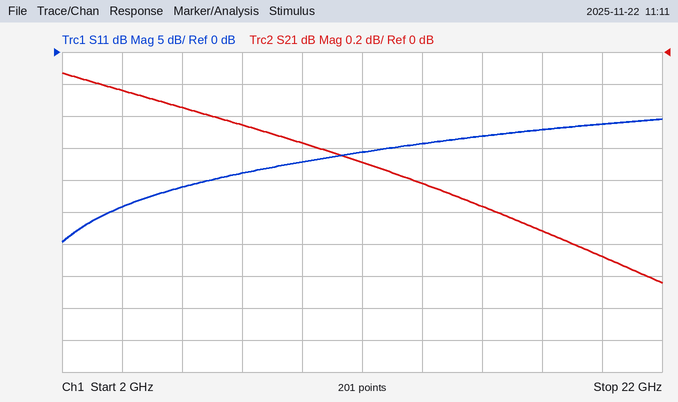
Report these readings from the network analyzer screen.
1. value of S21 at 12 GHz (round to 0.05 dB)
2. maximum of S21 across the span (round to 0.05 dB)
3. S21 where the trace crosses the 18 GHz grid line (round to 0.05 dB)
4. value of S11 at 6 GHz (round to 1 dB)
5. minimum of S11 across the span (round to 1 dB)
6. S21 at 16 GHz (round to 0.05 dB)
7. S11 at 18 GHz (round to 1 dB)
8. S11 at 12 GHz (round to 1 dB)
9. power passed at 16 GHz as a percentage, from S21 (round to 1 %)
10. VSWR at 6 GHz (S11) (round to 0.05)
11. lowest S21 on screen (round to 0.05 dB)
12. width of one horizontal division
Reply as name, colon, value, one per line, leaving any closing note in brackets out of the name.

value of S21 at 12 GHz: -0.70 dB
maximum of S21 across the span: -0.15 dB
S21 where the trace crosses the 18 GHz grid line: -1.10 dB
value of S11 at 6 GHz: -21 dB
minimum of S11 across the span: -30 dB
S21 at 16 GHz: -0.95 dB
S11 at 18 GHz: -12 dB
S11 at 12 GHz: -16 dB
power passed at 16 GHz as a percentage, from S21: 80 %
VSWR at 6 GHz (S11): 1.20
lowest S21 on screen: -1.45 dB
width of one horizontal division: 2 GHz
